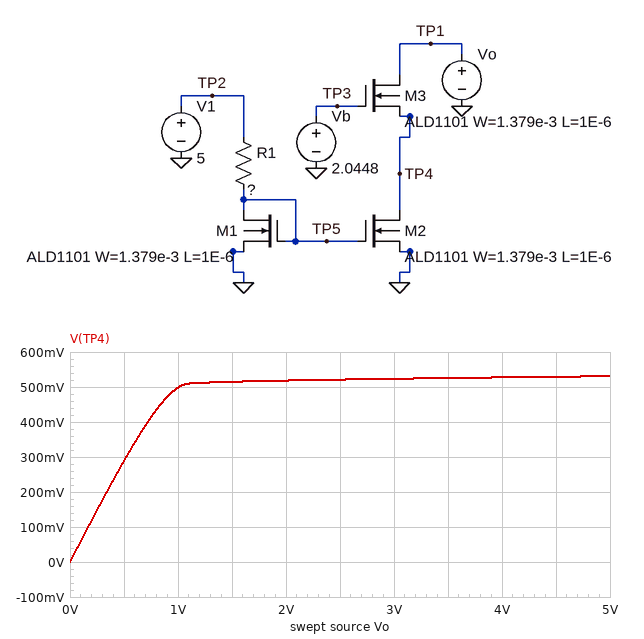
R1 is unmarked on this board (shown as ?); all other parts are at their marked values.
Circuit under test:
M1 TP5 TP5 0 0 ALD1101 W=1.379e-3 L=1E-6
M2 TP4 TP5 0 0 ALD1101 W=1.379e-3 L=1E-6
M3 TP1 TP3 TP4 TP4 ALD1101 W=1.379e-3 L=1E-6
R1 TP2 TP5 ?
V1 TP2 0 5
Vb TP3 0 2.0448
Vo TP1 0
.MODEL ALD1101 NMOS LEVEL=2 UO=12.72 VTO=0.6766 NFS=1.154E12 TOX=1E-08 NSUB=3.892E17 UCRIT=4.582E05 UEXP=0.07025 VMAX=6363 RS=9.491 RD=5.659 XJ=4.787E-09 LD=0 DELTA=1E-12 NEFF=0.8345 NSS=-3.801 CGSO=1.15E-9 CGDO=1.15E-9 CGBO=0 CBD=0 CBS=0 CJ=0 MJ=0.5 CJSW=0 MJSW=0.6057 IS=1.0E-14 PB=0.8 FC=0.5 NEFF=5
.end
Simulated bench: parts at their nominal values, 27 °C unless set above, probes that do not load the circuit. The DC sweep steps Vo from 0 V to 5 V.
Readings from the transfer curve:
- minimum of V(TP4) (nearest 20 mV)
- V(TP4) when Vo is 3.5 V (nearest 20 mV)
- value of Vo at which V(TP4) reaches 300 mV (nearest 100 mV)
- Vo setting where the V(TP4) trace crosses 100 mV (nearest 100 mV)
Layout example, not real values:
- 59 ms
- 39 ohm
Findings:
- 0 V
- 520 mV
- 500 mV
- 200 mV
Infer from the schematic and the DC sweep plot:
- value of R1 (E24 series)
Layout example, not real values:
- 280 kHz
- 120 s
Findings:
- 2.2 kΩ
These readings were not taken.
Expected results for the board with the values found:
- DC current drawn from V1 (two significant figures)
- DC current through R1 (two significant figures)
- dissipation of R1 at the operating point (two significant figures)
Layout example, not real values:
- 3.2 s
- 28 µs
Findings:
- 1.6 mA
- 1.6 mA
- 5.4 mW
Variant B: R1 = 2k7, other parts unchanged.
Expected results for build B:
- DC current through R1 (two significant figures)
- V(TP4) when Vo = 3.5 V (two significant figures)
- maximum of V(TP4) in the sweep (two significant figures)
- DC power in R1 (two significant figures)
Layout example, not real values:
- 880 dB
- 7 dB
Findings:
- 1.3 mA
- 590 mV
- 600 mV
- 4.6 mW
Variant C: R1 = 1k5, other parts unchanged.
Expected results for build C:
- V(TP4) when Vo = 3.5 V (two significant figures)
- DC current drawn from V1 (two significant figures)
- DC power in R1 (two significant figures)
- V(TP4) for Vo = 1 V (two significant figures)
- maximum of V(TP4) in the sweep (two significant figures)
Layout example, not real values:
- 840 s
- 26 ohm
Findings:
- 440 mV
- 2.2 mA
- 7.2 mW
- 420 mV
- 450 mV
